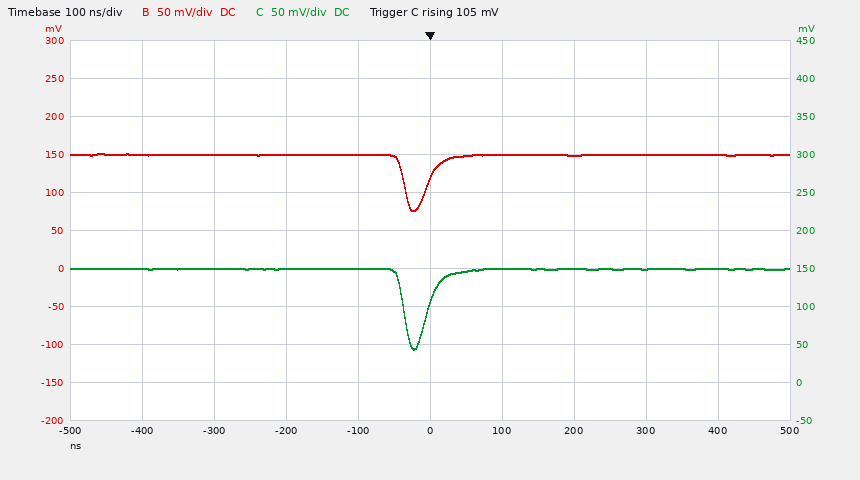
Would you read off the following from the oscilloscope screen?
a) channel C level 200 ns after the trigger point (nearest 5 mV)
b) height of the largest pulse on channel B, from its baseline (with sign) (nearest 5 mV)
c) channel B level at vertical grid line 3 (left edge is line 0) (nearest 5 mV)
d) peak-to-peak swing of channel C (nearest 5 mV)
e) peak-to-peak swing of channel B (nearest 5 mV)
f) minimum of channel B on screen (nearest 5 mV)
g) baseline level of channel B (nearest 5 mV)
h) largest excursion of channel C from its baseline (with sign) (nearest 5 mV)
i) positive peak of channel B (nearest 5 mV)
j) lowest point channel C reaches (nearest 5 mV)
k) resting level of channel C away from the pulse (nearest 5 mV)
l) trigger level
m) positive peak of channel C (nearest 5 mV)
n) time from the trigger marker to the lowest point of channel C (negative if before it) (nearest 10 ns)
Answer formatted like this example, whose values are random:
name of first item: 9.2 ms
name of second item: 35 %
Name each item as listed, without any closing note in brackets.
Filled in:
channel C level 200 ns after the trigger point: 150 mV
height of the largest pulse on channel B, from its baseline (with sign): -75 mV
channel B level at vertical grid line 3 (left edge is line 0): 150 mV
peak-to-peak swing of channel C: 105 mV
peak-to-peak swing of channel B: 75 mV
minimum of channel B on screen: 75 mV
baseline level of channel B: 150 mV
largest excursion of channel C from its baseline (with sign): -105 mV
positive peak of channel B: 150 mV
lowest point channel C reaches: 45 mV
resting level of channel C away from the pulse: 150 mV
trigger level: 105 mV
positive peak of channel C: 150 mV
time from the trigger marker to the lowest point of channel C (negative if before it): -20 ns
